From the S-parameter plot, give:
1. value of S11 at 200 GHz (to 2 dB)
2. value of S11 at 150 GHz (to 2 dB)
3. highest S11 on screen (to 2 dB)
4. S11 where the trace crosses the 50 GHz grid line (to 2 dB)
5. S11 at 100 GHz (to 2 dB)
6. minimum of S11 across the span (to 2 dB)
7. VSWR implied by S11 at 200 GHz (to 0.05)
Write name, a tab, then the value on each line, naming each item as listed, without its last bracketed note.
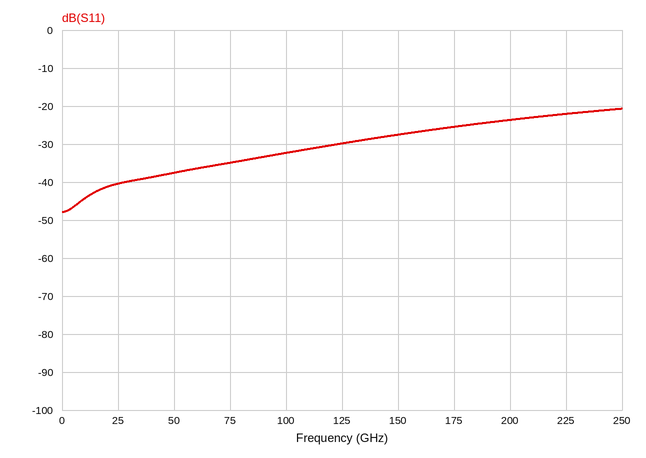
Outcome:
value of S11 at 200 GHz	-24 dB
value of S11 at 150 GHz	-28 dB
highest S11 on screen	-20 dB
S11 where the trace crosses the 50 GHz grid line	-38 dB
S11 at 100 GHz	-32 dB
minimum of S11 across the span	-48 dB
VSWR implied by S11 at 200 GHz	1.15
